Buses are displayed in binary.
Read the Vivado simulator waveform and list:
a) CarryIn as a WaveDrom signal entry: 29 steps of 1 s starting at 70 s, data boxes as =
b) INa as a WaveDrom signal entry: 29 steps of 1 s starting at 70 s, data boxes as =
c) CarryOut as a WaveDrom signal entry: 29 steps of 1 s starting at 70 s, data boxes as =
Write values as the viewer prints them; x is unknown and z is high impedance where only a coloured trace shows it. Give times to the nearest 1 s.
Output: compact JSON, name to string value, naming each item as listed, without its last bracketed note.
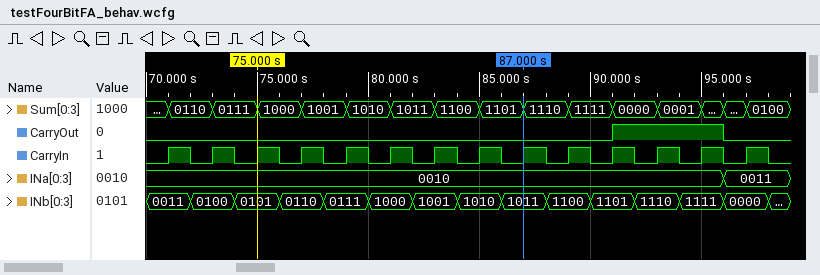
{"CarryIn as a WaveDrom signal entry: 29 steps of 1 s starting at 70 s, data boxes as =": "{name: 'CarryIn', wave: '01010101010101010101010101010'}", "INa as a WaveDrom signal entry: 29 steps of 1 s starting at 70 s, data boxes as =": "{name: 'INa', wave: '=.........................=..', data: '0010 0011'}", "CarryOut as a WaveDrom signal entry: 29 steps of 1 s starting at 70 s, data boxes as =": "{name: 'CarryOut', wave: '0....................1....0..'}"}
